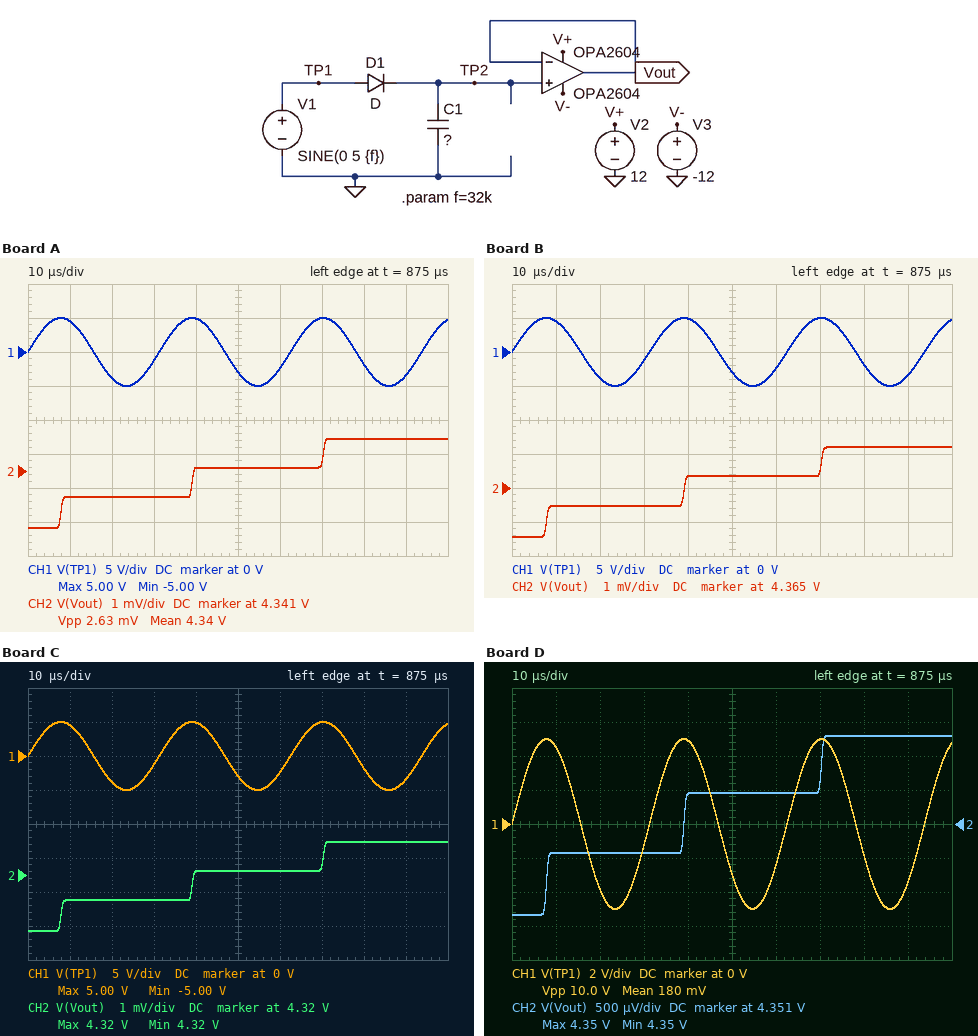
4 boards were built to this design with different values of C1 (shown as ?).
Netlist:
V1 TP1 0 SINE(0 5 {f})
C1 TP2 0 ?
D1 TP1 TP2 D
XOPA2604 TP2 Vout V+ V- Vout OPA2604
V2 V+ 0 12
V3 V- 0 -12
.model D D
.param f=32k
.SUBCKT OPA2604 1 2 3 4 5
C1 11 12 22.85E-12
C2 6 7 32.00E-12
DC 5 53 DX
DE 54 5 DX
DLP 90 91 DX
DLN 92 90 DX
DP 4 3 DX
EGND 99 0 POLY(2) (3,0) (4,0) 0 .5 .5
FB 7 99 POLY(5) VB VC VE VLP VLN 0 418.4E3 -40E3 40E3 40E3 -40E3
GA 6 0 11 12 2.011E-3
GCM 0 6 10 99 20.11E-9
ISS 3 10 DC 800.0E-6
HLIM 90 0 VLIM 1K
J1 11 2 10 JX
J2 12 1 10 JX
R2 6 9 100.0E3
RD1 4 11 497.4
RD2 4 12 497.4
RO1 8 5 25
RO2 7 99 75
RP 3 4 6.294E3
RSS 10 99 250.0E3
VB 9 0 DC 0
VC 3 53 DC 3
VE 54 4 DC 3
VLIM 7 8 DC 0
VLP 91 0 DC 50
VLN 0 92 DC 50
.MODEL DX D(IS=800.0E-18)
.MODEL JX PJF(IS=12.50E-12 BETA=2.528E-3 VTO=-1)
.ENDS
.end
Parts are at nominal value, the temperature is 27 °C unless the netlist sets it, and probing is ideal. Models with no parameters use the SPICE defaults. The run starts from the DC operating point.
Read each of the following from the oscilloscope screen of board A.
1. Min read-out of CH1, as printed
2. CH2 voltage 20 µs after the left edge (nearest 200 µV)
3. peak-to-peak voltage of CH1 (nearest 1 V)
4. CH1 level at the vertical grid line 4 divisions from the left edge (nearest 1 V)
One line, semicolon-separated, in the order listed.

-5.00 V; 4.3402 V; 10 V; 5 V
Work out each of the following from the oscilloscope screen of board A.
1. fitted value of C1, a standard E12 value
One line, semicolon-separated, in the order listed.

1.2 µF
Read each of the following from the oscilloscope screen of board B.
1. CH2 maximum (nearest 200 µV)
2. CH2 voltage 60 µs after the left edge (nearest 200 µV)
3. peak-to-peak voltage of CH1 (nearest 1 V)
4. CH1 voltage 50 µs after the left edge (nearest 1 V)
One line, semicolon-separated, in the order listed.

4.3662 V; 4.3654 V; 10 V; -3 V
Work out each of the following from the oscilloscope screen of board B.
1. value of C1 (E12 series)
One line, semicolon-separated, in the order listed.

470 nF
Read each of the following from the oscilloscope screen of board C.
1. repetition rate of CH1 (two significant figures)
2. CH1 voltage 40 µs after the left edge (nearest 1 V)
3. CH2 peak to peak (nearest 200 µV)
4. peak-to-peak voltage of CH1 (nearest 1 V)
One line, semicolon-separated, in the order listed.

32 kHz; 5 V; 2.6 mV; 10 V
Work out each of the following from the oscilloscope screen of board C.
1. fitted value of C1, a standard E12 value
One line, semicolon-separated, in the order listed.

2.7 µF
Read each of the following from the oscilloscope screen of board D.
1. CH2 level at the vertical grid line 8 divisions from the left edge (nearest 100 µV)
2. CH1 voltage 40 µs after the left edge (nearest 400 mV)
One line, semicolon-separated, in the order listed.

4.3518 V; 4.8 V
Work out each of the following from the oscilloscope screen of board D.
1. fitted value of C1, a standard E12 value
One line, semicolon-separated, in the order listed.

820 nF
